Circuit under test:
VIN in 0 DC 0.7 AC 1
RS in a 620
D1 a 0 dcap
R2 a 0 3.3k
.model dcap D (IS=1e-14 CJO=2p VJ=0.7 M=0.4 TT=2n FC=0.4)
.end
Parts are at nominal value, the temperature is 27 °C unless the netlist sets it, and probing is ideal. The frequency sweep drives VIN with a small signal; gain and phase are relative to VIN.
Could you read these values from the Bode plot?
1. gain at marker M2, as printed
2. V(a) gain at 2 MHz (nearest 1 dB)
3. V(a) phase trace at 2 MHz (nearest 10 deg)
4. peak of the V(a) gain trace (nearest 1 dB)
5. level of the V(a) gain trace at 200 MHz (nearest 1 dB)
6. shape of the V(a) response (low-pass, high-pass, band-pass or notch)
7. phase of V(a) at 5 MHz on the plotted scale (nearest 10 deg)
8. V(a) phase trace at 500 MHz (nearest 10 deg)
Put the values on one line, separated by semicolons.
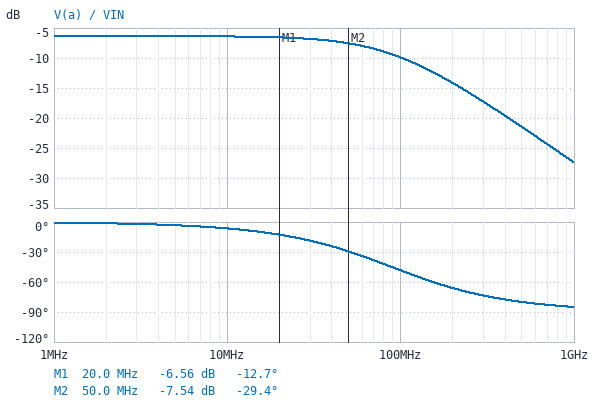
-7.54 dB; -6 dB; 0 deg; -6 dB; -14 dB; low-pass; 0 deg; -80 deg
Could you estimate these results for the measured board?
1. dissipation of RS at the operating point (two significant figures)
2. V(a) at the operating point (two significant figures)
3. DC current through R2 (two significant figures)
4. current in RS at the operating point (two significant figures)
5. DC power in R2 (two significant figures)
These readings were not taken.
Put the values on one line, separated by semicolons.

27 µW; 570 mV; 170 µA; 210 µA; 98 µW
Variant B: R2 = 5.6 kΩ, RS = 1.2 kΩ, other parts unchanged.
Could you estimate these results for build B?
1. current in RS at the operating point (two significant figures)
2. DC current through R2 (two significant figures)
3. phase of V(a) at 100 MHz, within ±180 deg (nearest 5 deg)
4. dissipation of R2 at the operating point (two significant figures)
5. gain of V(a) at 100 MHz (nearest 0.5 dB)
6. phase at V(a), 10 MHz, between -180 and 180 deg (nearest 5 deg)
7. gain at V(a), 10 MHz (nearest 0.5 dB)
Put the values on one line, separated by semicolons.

120 µA; 99 µA; -60 deg; 55 µW; -12.5 dB; -10 deg; -7.0 dB
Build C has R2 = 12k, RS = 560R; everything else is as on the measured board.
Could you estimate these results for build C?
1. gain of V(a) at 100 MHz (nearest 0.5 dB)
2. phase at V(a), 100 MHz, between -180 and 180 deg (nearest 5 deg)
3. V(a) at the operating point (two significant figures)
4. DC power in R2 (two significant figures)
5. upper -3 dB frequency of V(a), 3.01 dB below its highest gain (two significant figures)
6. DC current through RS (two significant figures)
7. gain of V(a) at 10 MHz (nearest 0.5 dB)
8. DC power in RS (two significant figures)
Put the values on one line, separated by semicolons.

-15.5 dB; -50 deg; 600 mV; 30 µW; 83 MHz; 180 µA; -11.5 dB; 17 µW
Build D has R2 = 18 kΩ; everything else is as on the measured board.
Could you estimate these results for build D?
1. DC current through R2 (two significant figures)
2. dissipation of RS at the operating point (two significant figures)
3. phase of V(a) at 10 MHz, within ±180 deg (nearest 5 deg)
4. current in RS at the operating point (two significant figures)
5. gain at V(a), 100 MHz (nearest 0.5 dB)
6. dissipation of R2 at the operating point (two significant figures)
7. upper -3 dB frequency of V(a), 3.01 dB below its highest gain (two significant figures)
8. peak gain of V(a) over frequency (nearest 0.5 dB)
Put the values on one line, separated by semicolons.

33 µA; 16 µW; -5 deg; 160 µA; -16.0 dB; 20 µW; 80 MHz; -12.0 dB
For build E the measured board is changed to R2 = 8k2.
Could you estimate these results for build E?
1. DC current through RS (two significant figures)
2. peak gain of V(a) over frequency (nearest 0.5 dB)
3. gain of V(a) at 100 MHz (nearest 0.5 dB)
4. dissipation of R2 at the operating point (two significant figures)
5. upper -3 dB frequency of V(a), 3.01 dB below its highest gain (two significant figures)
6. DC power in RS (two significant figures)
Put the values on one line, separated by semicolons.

170 µA; -10.5 dB; -14.5 dB; 43 µW; 82 MHz; 18 µW
